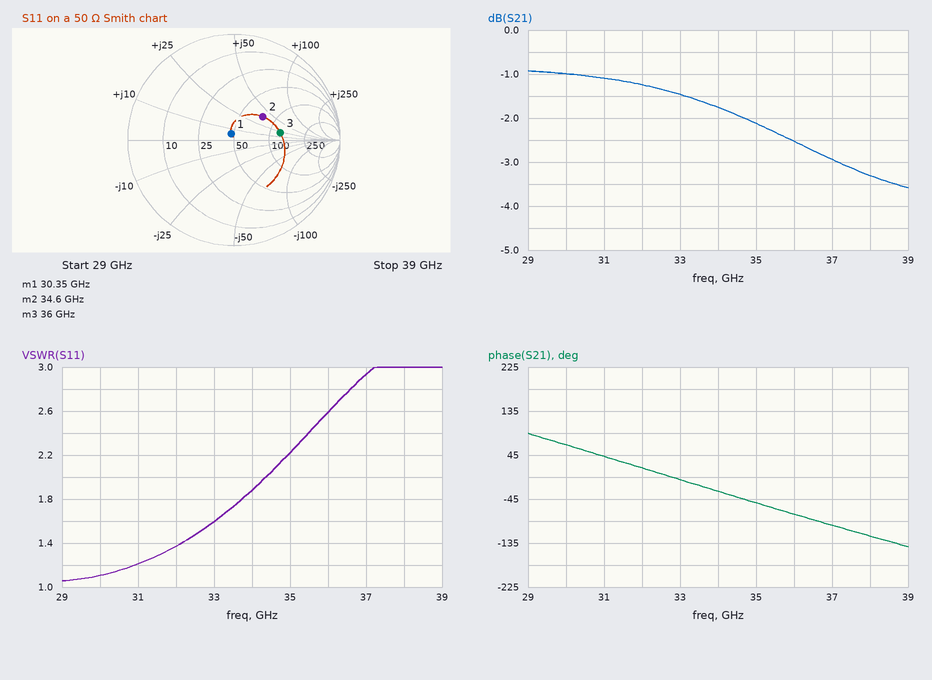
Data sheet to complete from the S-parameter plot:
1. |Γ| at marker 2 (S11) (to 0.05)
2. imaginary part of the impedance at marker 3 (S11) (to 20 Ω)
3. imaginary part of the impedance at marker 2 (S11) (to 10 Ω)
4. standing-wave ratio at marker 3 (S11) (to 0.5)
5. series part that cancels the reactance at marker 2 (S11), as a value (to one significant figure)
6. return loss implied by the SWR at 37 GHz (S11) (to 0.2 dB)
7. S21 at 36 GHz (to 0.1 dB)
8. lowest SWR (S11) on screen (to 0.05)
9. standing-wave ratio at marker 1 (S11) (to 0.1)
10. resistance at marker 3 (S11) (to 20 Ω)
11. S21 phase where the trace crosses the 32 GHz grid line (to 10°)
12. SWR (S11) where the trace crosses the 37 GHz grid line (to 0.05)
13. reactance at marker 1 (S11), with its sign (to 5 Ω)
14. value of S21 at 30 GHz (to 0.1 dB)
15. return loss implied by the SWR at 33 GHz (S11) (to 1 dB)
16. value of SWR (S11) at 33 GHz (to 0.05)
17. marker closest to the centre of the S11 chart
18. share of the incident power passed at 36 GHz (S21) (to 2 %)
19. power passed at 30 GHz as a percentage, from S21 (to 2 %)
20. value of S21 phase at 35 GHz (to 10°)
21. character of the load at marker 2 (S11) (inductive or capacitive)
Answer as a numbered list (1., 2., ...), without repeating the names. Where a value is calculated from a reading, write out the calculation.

1. 0.35
2. +20 Ω
3. +40 Ω
4. 2.5
5. C = 1/(2π × 34.6 GHz × 40 Ω) ≈ 115 fF, so 100 fF to one significant figure
6. −20 log10((2.95 − 1)/(2.95 + 1)) ≈ 6.13 dB, so 6.2 dB to the nearest 0.2 dB
7. -2.5 dB
8. 1.05
9. 1.1
10. 120 Ω
11. 20°
12. 2.95
13. +5 Ω
14. -1.0 dB
15. −20 log10((1.6 − 1)/(1.6 + 1)) ≈ 13 dB
16. 1.60
17. marker 1
18. 10^(-2.5/10) ≈ 56 %
19. 10^(-1/10) ≈ 79.4 %, so 80 % to the nearest 2 %
20. -50°
21. inductive
